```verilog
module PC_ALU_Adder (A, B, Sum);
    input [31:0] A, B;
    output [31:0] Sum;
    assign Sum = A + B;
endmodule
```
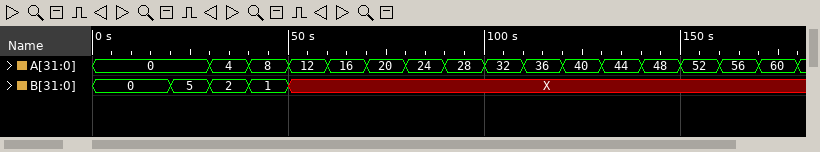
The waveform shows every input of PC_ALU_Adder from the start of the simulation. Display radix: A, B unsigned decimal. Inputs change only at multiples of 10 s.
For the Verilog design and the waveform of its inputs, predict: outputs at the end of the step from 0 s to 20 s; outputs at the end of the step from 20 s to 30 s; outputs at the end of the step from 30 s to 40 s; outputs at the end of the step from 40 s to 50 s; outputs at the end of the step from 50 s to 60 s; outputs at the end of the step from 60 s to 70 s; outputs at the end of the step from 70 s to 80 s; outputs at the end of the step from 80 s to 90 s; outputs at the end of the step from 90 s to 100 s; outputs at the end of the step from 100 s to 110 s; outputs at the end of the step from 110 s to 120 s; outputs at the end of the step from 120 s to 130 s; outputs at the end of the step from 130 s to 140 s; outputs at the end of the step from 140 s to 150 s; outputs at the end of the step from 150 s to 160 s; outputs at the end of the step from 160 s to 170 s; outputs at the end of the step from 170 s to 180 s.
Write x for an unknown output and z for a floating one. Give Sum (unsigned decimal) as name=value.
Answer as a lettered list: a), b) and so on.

a) Sum=0
b) Sum=5
c) Sum=6
d) Sum=9
e) Sum=x
f) Sum=x
g) Sum=x
h) Sum=x
i) Sum=x
j) Sum=x
k) Sum=x
l) Sum=x
m) Sum=x
n) Sum=x
o) Sum=x
p) Sum=x
q) Sum=x
